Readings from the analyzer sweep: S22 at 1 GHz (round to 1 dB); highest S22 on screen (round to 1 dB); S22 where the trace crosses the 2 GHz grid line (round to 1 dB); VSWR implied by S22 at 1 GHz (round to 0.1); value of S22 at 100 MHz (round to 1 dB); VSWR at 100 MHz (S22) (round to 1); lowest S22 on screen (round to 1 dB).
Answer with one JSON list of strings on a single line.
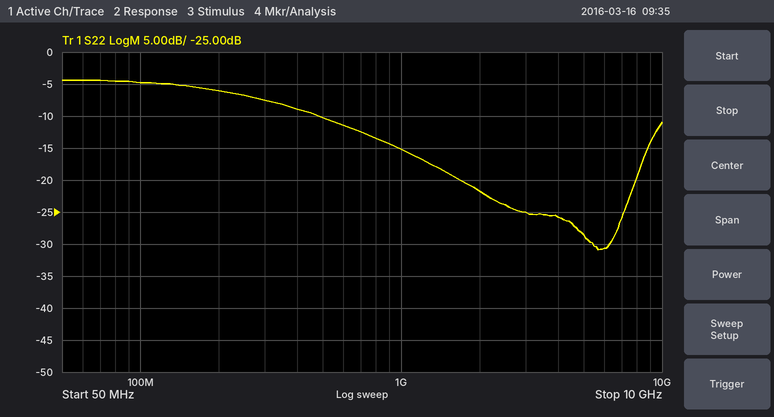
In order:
["-15 dB", "-4 dB", "-22 dB", "1.4", "-5 dB", "4", "-31 dB"]
